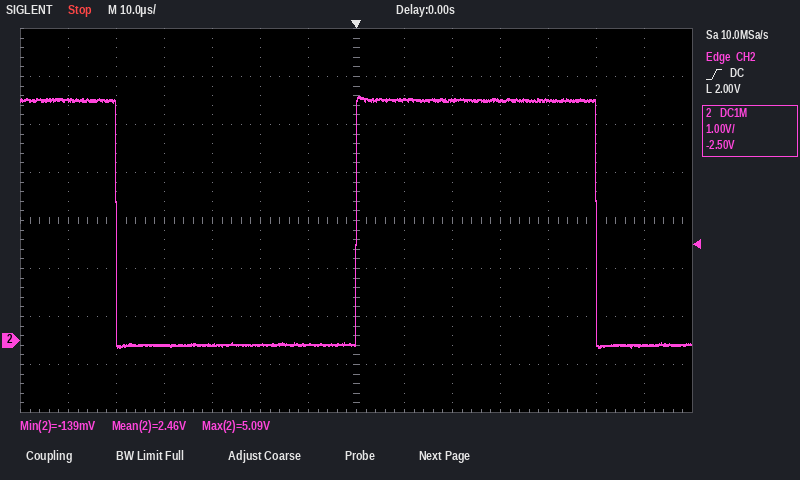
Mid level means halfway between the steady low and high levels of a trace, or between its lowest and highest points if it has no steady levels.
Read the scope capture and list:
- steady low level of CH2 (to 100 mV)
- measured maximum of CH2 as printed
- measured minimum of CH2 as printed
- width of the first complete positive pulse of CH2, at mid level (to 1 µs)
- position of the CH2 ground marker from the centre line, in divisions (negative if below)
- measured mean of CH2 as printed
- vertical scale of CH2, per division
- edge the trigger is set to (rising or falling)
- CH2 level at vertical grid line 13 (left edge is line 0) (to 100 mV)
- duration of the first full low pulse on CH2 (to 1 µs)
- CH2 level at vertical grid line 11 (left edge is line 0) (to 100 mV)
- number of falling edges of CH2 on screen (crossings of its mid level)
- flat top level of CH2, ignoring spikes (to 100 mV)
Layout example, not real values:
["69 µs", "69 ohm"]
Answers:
["-100 mV", "5.09 V", "-139 mV", "50 µs", "-2.5 div", "2.46 V", "1 V", "rising", "-100 mV", "50 µs", "5.0 V", "2", "5.0 V"]
